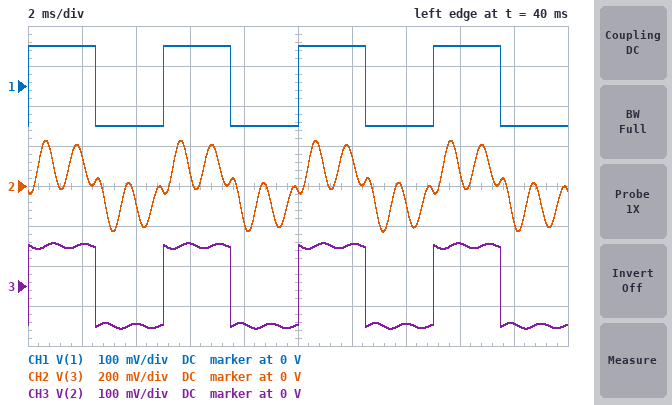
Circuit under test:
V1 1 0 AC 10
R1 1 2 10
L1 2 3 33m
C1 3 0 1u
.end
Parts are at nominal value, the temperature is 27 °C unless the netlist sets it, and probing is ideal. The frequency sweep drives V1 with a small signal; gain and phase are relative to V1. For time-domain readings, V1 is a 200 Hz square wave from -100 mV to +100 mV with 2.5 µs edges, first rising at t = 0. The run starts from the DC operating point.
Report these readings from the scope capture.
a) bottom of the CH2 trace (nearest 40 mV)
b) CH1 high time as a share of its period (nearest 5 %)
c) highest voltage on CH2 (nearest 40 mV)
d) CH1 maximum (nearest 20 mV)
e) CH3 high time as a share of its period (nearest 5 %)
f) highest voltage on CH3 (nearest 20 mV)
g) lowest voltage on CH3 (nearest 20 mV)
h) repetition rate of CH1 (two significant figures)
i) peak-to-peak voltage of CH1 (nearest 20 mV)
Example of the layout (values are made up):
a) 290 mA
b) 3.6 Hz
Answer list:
a) -240 mV
b) 50 %
c) 240 mV
d) 100 mV
e) 50 %
f) 100 mV
g) -100 mV
h) 200 Hz
i) 200 mV
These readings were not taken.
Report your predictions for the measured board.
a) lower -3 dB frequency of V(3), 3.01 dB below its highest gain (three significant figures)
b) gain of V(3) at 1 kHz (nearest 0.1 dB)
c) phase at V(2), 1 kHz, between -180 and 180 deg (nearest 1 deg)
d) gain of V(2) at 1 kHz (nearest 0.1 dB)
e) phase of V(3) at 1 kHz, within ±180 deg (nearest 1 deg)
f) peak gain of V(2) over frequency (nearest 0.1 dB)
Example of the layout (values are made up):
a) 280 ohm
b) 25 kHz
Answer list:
a) 851 Hz
b) 10.2 dB
c) 12 deg
d) -0.2 dB
e) -168 deg
f) 0 dB
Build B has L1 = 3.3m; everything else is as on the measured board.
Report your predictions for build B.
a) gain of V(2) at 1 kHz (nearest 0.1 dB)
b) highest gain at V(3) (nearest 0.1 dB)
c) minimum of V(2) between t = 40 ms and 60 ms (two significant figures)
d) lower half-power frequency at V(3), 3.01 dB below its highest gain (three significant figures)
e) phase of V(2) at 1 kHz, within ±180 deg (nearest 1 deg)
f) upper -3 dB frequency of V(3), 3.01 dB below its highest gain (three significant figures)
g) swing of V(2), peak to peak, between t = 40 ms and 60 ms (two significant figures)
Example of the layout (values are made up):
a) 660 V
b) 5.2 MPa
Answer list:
a) 0 dB
b) 15.2 dB
c) -120 mV
d) 2.50 kHz
e) -4 deg
f) 2.98 kHz
g) 250 mV
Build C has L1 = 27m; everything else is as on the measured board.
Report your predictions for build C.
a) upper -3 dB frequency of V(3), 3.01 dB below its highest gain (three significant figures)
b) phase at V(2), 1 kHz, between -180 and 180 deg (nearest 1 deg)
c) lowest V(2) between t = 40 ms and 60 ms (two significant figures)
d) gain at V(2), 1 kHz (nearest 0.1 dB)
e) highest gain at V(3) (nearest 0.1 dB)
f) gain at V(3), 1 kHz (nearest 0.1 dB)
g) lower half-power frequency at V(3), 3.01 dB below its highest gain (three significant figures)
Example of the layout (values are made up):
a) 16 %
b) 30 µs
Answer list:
a) 997 Hz
b) 44 deg
c) -120 mV
d) -2.8 dB
e) 24.3 dB
f) 20.8 dB
g) 938 Hz
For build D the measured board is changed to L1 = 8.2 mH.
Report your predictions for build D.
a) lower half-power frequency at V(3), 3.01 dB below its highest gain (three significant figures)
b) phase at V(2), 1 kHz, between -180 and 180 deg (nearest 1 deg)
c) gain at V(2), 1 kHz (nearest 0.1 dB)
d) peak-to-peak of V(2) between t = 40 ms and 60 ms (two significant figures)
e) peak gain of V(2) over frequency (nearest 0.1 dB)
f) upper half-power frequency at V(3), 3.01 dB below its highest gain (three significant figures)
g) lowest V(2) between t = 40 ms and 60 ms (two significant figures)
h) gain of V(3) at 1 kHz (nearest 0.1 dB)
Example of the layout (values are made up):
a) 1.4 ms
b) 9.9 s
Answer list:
a) 1.65 kHz
b) -5 deg
c) 0 dB
d) 240 mV
e) 0 dB
f) 1.85 kHz
g) -120 mV
h) 3.4 dB
